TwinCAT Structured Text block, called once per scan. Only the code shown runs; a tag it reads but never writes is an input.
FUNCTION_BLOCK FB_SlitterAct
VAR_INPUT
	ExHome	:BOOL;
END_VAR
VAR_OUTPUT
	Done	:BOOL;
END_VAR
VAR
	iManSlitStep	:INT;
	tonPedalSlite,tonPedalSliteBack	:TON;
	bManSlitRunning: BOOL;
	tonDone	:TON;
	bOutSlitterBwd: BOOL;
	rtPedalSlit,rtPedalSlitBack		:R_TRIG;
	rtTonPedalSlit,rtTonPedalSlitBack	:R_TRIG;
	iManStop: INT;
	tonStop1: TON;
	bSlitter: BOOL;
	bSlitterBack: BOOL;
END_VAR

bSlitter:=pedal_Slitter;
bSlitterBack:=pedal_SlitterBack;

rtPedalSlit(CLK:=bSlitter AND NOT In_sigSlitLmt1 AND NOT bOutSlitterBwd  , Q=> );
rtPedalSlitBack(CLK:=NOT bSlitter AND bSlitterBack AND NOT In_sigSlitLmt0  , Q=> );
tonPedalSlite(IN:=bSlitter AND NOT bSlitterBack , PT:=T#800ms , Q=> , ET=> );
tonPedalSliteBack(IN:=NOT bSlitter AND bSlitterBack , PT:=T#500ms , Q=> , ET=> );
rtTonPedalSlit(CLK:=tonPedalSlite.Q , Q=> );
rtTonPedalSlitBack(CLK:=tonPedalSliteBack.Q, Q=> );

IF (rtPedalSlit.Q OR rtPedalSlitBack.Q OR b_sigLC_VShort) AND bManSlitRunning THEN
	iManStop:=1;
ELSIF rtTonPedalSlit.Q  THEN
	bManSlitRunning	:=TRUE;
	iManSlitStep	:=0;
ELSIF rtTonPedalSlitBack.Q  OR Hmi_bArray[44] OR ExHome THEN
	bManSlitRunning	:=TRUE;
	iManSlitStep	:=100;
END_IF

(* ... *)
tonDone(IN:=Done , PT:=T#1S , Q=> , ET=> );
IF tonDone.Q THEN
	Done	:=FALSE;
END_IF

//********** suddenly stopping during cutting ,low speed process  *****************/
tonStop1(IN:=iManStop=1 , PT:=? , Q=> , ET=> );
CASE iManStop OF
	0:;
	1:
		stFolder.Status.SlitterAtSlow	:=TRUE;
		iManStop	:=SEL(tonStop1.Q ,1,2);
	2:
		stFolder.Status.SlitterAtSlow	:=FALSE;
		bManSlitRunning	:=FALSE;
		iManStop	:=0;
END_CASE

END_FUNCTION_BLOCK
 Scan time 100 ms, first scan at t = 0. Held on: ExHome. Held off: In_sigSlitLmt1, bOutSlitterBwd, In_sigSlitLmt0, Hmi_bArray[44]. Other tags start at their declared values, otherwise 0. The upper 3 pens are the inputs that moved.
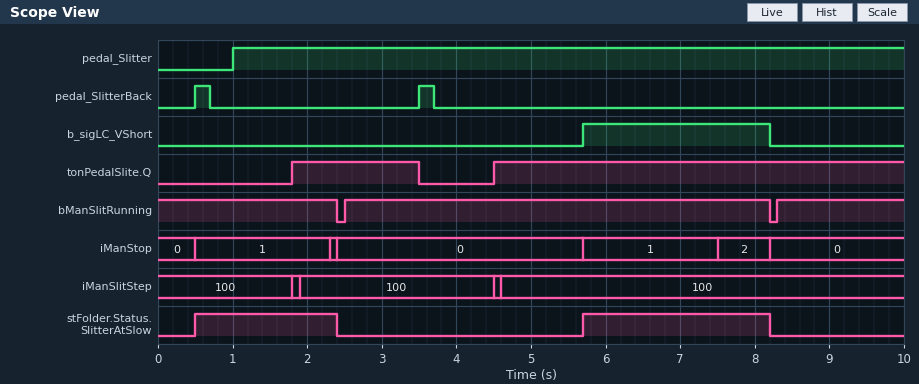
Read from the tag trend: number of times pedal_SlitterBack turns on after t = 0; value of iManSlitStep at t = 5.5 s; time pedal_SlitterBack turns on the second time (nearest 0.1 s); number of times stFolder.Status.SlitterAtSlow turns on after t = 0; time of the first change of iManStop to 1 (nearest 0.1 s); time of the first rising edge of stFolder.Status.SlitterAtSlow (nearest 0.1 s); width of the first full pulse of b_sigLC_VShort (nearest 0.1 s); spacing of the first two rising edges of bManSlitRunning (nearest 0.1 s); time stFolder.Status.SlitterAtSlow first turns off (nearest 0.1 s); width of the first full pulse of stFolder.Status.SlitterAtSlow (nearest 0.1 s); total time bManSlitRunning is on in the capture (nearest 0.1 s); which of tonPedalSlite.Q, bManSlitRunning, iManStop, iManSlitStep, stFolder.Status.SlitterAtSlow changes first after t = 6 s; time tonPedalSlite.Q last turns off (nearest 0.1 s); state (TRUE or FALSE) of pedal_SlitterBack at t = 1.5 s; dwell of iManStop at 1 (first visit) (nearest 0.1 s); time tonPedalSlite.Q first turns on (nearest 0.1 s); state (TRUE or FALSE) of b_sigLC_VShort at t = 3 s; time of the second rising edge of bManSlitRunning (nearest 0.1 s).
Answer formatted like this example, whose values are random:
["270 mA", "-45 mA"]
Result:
["2", "100", "3.5 s", "2", "0.5 s", "0.5 s", "2.5 s", "5.8 s", "2.4 s", "1.9 s", "9.8 s", "iManStop", "3.5 s", "FALSE", "1.8 s", "1.8 s", "FALSE", "8.3 s"]
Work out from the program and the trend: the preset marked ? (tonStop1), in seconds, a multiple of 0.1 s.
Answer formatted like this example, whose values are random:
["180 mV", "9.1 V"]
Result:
["1.8 s"]
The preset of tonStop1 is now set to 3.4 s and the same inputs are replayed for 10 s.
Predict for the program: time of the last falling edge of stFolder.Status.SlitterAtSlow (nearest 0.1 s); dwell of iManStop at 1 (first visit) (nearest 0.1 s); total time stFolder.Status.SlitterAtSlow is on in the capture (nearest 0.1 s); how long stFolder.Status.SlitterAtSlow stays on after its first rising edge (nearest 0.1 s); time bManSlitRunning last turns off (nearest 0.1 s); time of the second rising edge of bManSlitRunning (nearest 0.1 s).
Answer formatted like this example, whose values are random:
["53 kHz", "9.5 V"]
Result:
["9.2 s", "3.4 s", "7.0 s", "3.5 s", "9.2 s", "9.3 s"]
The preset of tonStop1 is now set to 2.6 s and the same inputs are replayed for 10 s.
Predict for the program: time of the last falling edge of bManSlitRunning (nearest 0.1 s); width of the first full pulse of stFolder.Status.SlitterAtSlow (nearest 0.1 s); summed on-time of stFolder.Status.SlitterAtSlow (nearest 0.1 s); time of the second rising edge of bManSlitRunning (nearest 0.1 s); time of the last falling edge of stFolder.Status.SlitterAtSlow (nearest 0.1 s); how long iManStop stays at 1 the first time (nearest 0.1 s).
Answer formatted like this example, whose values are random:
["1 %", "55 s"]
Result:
["8.4 s", "2.7 s", "5.4 s", "8.5 s", "8.4 s", "2.6 s"]
